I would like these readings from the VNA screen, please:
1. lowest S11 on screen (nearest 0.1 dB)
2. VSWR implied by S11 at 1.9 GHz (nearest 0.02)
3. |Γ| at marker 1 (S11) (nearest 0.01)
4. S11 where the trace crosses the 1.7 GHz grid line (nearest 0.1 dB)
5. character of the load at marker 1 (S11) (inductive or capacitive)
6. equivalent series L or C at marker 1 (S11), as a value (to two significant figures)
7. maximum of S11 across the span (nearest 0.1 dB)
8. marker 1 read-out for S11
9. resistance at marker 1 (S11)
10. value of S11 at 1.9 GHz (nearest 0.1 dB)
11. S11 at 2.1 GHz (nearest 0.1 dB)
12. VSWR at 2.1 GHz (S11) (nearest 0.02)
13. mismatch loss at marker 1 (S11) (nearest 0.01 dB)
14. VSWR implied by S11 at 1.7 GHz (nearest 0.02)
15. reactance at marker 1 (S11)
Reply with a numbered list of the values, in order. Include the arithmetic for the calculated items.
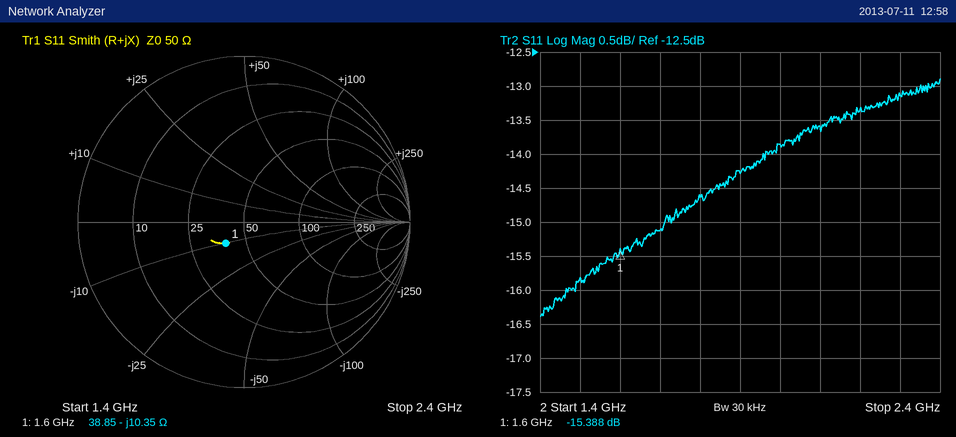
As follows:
1. -16.4 dB
2. |Γ| = 10^(-14.3/20) = 0.1928; VSWR = (1 + 0.1928)/(1 − 0.1928) ≈ 1.48
3. 0.17
4. -15.1 dB
5. capacitive
6. C = 1/(2π × 1.6 GHz × 10.35 Ω) ≈ 9.6 pF
7. -12.9 dB
8. -15.388 dB
9. 38.85 Ω
10. -14.3 dB
11. -13.6 dB
12. |Γ| = 10^(-13.6/20) = 0.2089; VSWR = (1 + 0.2089)/(1 − 0.2089) ≈ 1.53, so 1.52 to the nearest 0.02
13. −10 log10(1 − 10^(-15.388/10)) ≈ 0.13 dB
14. |Γ| = 10^(-15.1/20) = 0.1758; VSWR = (1 + 0.1758)/(1 − 0.1758) ≈ 1.43, so 1.42 to the nearest 0.02
15. -10.35 Ω
